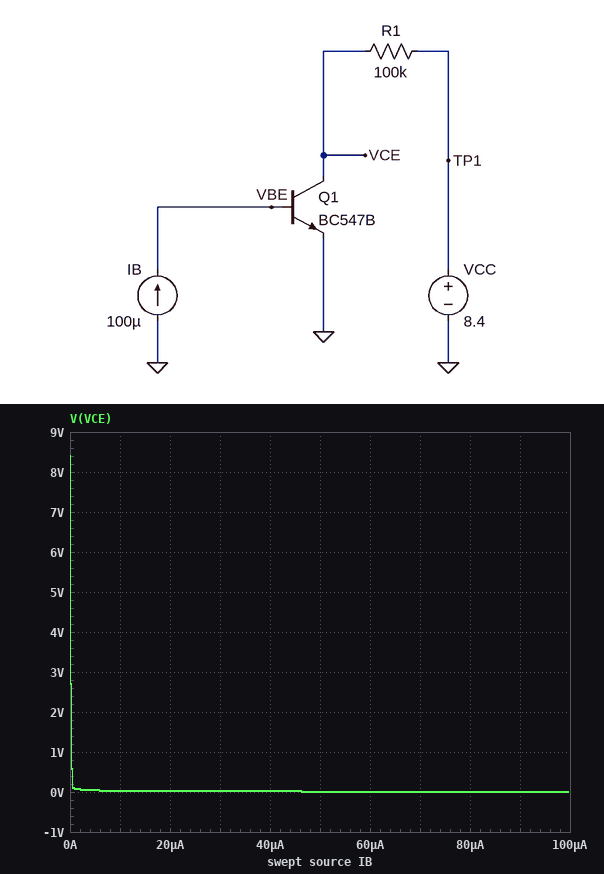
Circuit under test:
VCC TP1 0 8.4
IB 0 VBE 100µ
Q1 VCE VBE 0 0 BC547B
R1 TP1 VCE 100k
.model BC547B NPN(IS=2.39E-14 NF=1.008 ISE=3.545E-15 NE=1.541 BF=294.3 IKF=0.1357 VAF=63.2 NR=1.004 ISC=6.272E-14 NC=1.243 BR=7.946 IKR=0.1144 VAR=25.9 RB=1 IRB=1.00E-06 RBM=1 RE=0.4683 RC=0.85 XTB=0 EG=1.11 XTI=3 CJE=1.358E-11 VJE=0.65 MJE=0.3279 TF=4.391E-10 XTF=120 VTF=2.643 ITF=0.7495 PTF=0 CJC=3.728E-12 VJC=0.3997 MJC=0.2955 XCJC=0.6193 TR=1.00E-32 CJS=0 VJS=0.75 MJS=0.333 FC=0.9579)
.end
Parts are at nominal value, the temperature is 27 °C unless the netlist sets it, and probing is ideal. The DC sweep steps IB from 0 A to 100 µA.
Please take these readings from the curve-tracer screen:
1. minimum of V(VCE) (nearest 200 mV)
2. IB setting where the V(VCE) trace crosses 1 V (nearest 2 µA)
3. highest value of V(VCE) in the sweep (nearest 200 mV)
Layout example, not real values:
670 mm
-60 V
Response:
0 V
0 A
8.4 V
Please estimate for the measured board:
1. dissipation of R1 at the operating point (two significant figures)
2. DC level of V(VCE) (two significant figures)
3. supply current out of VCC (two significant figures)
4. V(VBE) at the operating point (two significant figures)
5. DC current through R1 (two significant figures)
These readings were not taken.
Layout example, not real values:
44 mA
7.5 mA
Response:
700 µW
9.4 mV
84 µA
630 mV
84 µA
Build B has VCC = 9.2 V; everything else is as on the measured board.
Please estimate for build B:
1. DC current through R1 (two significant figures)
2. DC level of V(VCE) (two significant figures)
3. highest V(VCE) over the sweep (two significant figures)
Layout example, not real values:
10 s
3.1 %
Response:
92 µA
9.7 mV
9.2 V
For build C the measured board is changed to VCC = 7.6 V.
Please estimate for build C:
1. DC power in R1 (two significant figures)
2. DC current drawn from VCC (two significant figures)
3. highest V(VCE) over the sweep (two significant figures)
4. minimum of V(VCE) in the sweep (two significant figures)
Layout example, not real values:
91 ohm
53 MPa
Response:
580 µW
76 µA
7.6 V
9.1 mV
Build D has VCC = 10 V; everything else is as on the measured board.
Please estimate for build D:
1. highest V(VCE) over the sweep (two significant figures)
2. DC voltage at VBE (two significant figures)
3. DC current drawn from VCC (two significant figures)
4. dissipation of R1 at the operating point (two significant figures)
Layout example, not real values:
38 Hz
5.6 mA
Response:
10 V
630 mV
100 µA
1.0 mW
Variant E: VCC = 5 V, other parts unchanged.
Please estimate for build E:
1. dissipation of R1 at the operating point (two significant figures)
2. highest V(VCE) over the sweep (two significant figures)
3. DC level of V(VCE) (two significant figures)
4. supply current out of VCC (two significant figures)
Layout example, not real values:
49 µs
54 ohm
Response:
250 µW
5.0 V
8.2 mV
50 µA
